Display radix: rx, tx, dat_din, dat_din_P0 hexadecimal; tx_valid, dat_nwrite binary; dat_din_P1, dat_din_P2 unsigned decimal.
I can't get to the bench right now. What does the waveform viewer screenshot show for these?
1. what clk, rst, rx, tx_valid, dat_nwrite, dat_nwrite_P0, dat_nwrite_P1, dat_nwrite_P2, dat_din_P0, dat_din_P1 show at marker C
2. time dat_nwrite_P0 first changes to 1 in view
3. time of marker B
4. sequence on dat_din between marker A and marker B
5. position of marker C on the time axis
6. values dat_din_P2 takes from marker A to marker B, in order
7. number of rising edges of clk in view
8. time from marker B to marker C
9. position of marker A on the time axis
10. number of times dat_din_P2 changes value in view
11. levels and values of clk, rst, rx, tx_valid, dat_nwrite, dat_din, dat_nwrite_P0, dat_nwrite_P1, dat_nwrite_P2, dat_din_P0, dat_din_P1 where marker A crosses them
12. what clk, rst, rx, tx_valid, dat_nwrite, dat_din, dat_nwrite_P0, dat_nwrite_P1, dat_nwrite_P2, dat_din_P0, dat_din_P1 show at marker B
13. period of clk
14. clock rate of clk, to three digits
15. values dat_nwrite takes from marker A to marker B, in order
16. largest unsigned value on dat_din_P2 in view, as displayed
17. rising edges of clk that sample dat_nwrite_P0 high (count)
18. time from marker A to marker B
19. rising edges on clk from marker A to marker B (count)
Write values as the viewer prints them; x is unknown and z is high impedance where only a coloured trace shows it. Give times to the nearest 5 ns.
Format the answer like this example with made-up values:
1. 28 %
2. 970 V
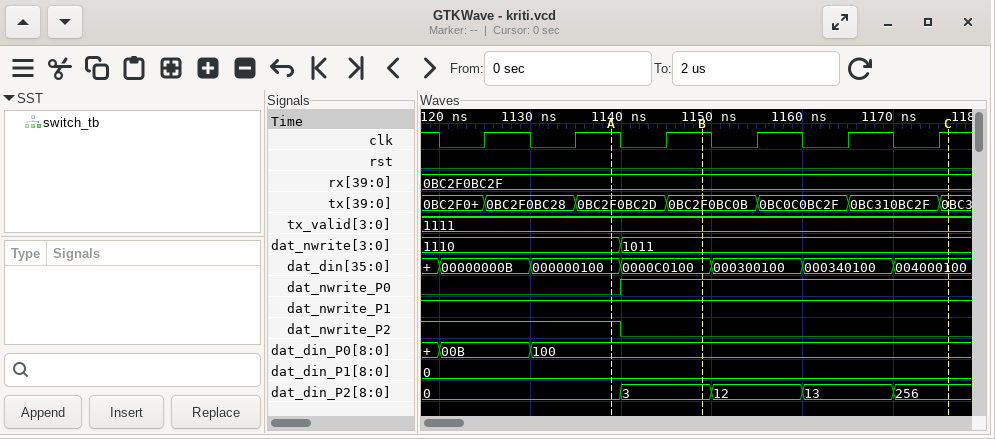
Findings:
1. clk=1, rst=0, rx=0BC2F0BC2F, tx_valid=1111, dat_nwrite=1011, dat_nwrite_P0=1, dat_nwrite_P1=1, dat_nwrite_P2=0, dat_din_P0=100, dat_din_P1=0
2. 1140 ns
3. 1150 ns
4. 000000100, 0000C0100
5. 1175 ns
6. 0, 3
7. 6
8. 25 ns
9. 1140 ns
10. 4
11. clk=1, rst=0, rx=0BC2F0BC2F, tx_valid=1111, dat_nwrite=1110, dat_din=000000100, dat_nwrite_P0=0, dat_nwrite_P1=1, dat_nwrite_P2=1, dat_din_P0=100, dat_din_P1=0
12. clk=1, rst=0, rx=0BC2F0BC2F, tx_valid=1111, dat_nwrite=1011, dat_din=0000C0100, dat_nwrite_P0=1, dat_nwrite_P1=1, dat_nwrite_P2=0, dat_din_P0=100, dat_din_P1=0
13. 10 ns
14. 100 MHz
15. 1110, 1011
16. 256
17. 4
18. 10 ns
19. 1
